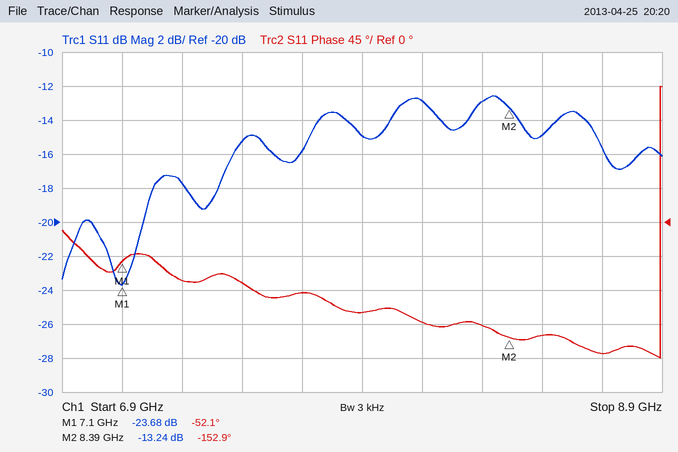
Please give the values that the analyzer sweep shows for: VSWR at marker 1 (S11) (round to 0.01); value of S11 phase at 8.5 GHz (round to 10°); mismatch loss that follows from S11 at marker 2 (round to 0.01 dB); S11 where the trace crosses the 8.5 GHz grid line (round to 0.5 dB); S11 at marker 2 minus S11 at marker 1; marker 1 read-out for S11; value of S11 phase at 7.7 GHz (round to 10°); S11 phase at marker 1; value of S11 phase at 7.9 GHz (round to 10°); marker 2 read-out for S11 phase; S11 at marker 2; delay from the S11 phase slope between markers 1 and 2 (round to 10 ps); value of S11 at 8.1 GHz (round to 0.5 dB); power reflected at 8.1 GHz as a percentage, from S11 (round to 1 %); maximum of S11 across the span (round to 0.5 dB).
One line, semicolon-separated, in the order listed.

1.14; -150°; 0.21 dB; -15.0 dB; 10.44 dB; -23.68 dB; -90°; -52.1°; -120°; -152.9°; -13.24 dB; 220 ps; -13.0 dB; 5 %; -12.5 dB
